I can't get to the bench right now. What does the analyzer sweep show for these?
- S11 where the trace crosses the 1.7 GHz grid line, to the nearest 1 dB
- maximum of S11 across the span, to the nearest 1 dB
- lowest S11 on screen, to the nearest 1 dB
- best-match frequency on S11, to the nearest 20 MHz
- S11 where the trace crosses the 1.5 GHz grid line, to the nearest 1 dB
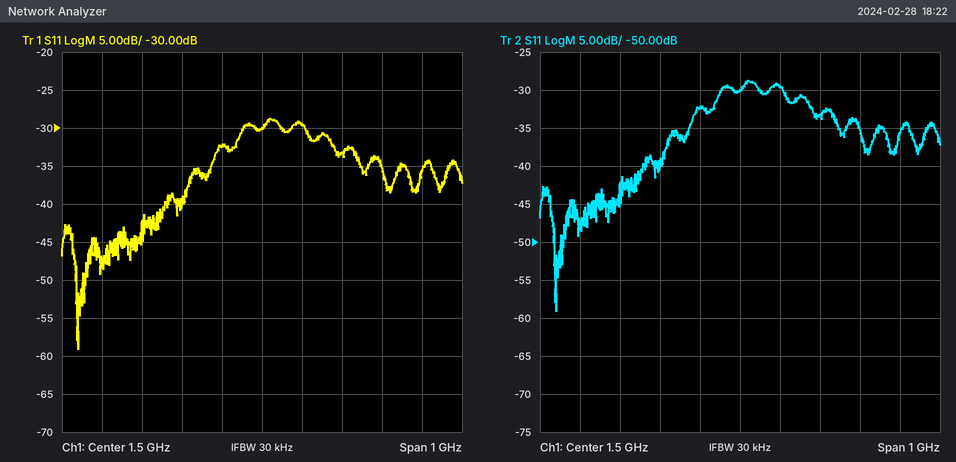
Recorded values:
-33 dB
-29 dB
-59 dB
1.04 GHz
-30 dB
